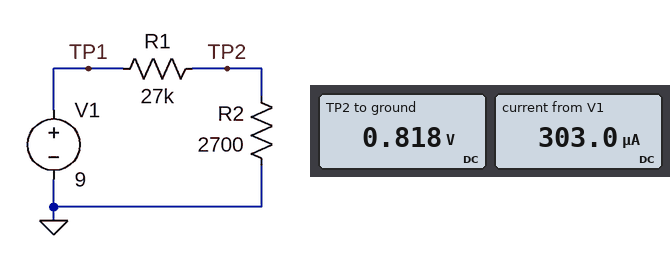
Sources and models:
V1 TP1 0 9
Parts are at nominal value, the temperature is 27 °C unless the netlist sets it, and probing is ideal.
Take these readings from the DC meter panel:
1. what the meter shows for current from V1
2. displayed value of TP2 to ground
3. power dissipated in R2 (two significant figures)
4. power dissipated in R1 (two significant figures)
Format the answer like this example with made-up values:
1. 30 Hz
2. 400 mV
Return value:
1. 303.0 µA
2. 0.818 V
3. 250 µW
4. 2.5 mW
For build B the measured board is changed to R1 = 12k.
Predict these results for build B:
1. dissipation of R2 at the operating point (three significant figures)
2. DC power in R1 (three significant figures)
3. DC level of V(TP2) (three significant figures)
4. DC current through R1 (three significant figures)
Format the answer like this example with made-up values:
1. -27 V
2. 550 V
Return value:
1. 1.01 mW
2. 4.50 mW
3. 1.65 V
4. 612 µA
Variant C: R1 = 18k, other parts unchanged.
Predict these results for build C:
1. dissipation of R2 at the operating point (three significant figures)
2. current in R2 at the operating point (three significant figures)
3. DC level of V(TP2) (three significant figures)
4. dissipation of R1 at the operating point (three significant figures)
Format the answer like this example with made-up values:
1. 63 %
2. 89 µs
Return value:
1. 510 µW
2. 435 µA
3. 1.17 V
4. 3.40 mW
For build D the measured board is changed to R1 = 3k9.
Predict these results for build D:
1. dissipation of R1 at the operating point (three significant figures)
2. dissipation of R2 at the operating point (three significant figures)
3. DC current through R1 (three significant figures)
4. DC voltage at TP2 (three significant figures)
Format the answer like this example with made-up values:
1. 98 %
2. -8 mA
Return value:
1. 7.25 mW
2. 5.02 mW
3. 1.36 mA
4. 3.68 V
